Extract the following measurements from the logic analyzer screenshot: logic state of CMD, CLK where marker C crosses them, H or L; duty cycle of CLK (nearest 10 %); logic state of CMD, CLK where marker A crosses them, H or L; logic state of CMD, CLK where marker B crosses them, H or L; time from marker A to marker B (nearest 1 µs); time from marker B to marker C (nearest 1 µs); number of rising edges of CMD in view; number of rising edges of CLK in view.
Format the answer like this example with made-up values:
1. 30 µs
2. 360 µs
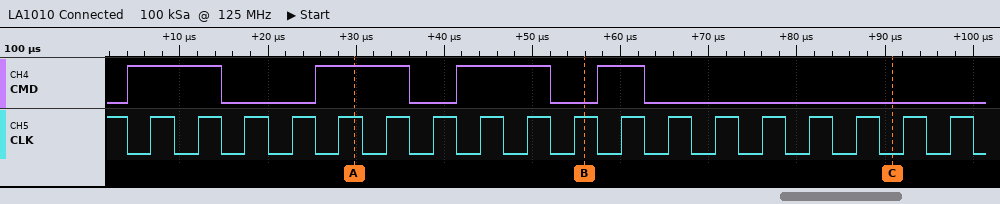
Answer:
1. CMD=L, CLK=L
2. 50 %
3. CMD=H, CLK=H
4. CMD=L, CLK=H
5. 26 µs
6. 35 µs
7. 4
8. 18
